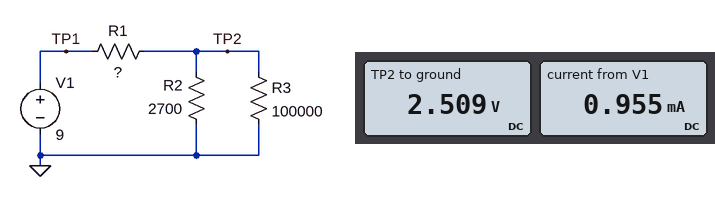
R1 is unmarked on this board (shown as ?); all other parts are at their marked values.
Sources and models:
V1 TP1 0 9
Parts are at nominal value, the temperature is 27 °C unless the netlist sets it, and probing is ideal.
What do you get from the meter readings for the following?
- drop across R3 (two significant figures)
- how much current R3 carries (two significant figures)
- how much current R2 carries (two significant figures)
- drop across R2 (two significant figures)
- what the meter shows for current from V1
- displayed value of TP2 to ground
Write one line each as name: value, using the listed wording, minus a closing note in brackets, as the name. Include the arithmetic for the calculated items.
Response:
drop across R3: 2.509 V = 2.5 V
how much current R3 carries: (2.509 V) / 100 kΩ = 25 µA
how much current R2 carries: (2.509 V) / 2.7 kΩ = 930 µA
drop across R2: 2.509 V = 2.5 V
what the meter shows for current from V1: 0.955 mA
displayed value of TP2 to ground: 2.509 V
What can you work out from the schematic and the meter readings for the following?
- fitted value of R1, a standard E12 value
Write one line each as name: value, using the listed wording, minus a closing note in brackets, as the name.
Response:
fitted value of R1, a standard E12 value: 6.8 kΩ
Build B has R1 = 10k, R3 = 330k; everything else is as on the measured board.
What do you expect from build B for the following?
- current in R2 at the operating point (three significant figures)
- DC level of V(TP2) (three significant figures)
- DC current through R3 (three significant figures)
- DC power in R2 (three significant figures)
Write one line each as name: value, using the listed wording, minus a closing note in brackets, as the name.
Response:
current in R2 at the operating point: 704 µA
DC level of V(TP2): 1.90 V
DC current through R3: 5.76 µA
DC power in R2: 1.34 mW
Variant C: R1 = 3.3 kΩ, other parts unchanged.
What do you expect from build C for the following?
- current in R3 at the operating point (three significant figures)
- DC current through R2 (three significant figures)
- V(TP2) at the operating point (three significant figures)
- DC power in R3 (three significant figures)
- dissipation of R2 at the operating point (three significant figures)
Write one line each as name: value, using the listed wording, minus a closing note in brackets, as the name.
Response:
current in R3 at the operating point: 39.9 µA
DC current through R2: 1.48 mA
V(TP2) at the operating point: 3.99 V
DC power in R3: 159 µW
dissipation of R2 at the operating point: 5.90 mW
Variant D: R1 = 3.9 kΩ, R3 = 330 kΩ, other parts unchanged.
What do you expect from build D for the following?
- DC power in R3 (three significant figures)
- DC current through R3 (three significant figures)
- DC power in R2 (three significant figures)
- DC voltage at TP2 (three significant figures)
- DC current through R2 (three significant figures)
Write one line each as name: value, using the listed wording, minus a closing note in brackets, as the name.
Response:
DC power in R3: 40.7 µW
DC current through R3: 11.1 µA
DC power in R2: 4.97 mW
DC voltage at TP2: 3.66 V
DC current through R2: 1.36 mA
